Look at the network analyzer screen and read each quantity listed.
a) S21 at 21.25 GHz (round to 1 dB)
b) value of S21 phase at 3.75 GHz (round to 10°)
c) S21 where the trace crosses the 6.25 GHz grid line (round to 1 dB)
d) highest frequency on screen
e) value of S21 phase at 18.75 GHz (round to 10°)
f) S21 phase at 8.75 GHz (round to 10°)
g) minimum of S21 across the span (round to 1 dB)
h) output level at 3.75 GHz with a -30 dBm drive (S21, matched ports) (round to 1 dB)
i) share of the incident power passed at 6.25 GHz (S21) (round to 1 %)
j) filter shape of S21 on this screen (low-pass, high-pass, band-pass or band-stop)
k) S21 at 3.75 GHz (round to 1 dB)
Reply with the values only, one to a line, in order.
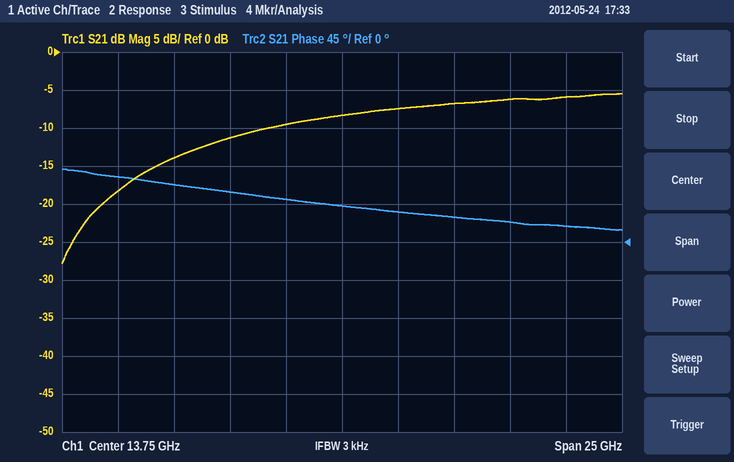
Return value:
-6 dB
80°
-14 dB
26.25 GHz
30°
60°
-28 dB
-48 dBm
4 %
high-pass
-18 dB
